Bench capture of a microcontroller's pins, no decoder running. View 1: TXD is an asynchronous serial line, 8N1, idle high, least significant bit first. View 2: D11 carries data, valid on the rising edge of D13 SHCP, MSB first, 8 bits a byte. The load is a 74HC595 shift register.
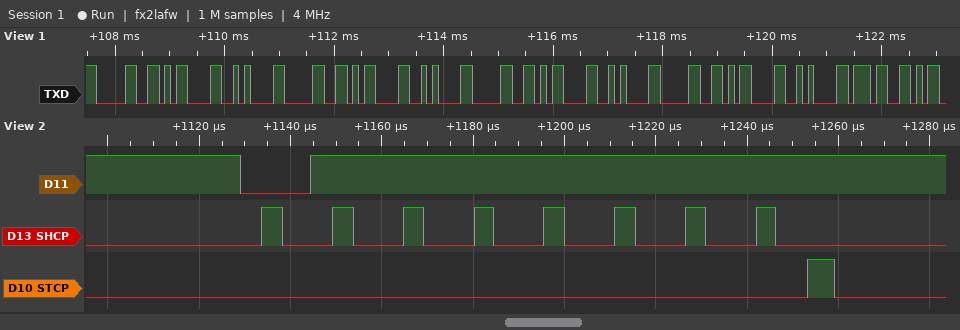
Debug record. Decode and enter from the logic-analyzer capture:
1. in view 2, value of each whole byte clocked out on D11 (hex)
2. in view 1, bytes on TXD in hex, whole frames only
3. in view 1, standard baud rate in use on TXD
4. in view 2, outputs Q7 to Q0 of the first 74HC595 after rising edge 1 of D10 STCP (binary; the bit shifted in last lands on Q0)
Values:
0x7F
30 0D 0A 30 0D 0A 30 0D 0A 30 0D 0A 37
9600 baud
01111111
